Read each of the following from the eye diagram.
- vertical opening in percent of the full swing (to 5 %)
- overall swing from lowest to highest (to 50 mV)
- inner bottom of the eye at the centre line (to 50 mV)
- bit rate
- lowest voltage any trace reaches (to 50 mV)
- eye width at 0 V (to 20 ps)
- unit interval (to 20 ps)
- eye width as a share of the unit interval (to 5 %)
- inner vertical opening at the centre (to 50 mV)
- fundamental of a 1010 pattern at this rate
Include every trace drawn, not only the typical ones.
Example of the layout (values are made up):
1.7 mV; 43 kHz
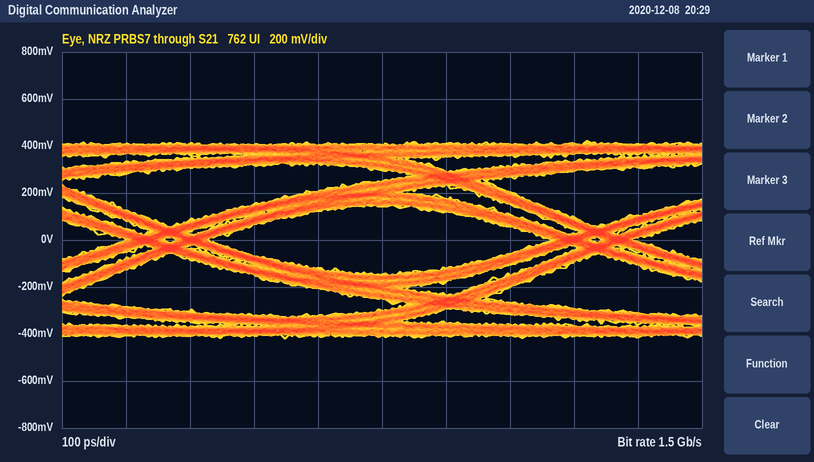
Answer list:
35 %; 850 mV; -150 mV; 1.5 Gb/s; -400 mV; 540 ps; 660 ps; 80 %; 300 mV; 750 MHz
